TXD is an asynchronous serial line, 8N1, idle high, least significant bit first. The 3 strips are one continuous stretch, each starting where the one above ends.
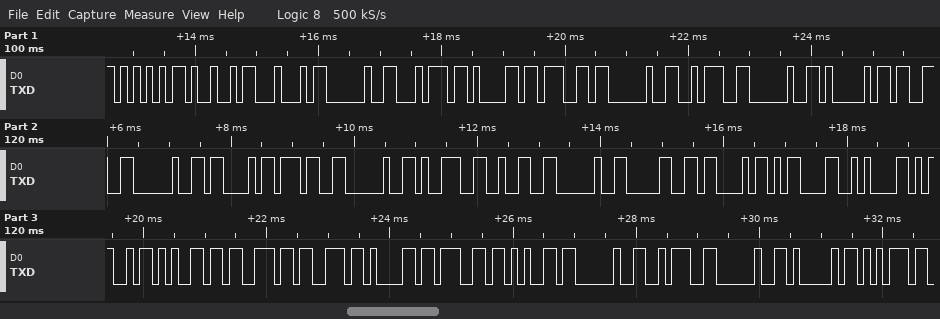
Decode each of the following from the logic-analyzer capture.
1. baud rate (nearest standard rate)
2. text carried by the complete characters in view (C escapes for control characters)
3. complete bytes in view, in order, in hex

9600 baud
"UID tag : A3 C7 92 0C\r\nMessage : Au"
55 49 44 20 74 61 67 20 3A 20 41 33 20 43 37 20 39 32 20 30 43 0D 0A 4D 65 73 73 61 67 65 20 3A 20 41 75
